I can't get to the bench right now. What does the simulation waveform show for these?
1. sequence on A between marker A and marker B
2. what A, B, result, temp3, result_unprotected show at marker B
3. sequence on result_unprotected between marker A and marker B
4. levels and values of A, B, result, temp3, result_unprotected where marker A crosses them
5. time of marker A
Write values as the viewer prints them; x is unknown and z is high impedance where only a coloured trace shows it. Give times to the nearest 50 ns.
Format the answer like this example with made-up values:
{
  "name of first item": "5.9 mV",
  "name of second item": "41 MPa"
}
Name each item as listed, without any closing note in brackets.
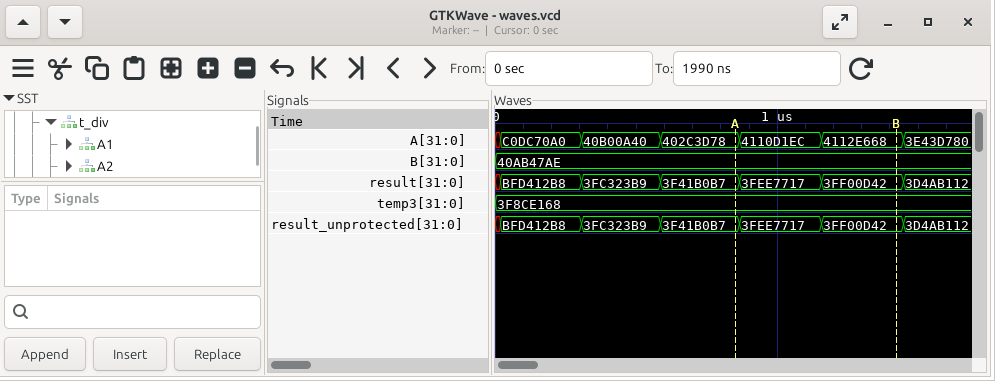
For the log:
{
  "sequence on A between marker A and marker B": "402C3D78, 4110D1EC, 4112E668",
  "what A, B, result, temp3, result_unprotected show at marker B": "A=4112E668, B=40AB47AE, result=3FF00D42, temp3=3F8CE168, result_unprotected=3FF00D42",
  "sequence on result_unprotected between marker A and marker B": "3F41B0B7, 3FEE7717, 3FF00D42",
  "levels and values of A, B, result, temp3, result_unprotected where marker A crosses them": "A=402C3D78, B=40AB47AE, result=3F41B0B7, temp3=3F8CE168, result_unprotected=3F41B0B7",
  "time of marker A": "850 ns"
}
